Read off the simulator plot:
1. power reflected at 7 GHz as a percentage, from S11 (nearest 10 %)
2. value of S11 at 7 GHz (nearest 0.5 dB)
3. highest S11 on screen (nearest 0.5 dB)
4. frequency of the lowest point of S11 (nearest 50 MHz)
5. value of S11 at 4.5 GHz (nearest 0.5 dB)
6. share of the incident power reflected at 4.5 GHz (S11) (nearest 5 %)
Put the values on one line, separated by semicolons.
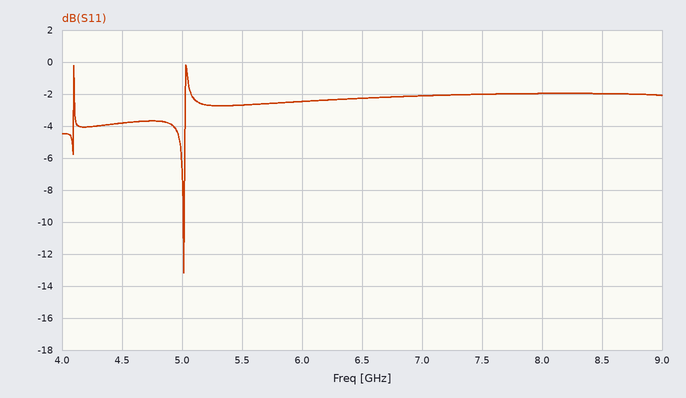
60 %; -2.0 dB; 0.0 dB; 5.00 GHz; -4.0 dB; 40 %
